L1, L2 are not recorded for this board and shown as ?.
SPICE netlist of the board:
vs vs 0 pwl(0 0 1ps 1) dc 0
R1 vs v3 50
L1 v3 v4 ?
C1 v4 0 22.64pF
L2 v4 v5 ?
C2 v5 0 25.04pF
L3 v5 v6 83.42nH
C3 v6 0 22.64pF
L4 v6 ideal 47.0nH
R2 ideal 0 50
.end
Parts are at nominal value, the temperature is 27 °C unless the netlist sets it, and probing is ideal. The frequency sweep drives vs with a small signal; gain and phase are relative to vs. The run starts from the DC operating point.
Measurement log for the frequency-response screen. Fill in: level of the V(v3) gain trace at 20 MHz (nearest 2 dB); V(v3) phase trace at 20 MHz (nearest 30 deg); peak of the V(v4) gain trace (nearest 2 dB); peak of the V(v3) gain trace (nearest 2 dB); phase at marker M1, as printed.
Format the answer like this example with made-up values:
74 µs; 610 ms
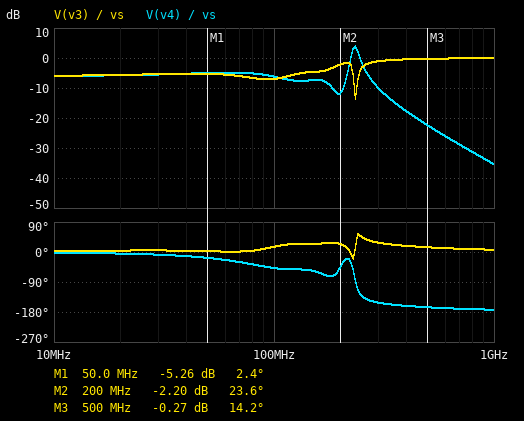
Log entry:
-6 dB; 0 deg; 4 dB; 0 dB; 2.4 deg
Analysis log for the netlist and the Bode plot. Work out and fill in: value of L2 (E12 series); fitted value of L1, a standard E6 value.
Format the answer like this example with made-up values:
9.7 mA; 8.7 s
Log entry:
56 nH; 68 nH
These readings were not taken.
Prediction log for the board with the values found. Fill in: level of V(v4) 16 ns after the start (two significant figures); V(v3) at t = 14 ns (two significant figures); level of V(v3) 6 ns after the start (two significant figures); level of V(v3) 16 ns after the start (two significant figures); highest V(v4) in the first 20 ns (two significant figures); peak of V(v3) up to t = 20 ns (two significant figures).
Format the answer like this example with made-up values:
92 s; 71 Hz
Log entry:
490 mV; 480 mV; 550 mV; 520 mV; 610 mV; 1.0 V
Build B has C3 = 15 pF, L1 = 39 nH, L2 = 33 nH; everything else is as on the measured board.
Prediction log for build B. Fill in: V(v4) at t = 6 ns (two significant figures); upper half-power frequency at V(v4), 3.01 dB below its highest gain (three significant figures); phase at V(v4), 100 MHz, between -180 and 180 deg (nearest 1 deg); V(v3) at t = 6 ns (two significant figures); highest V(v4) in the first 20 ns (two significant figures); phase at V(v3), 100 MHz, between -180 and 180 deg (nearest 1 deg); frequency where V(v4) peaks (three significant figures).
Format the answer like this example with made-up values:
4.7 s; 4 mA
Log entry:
540 mV; 306 MHz; -51 deg; 610 mV; 690 mV; -16 deg; 290 MHz
